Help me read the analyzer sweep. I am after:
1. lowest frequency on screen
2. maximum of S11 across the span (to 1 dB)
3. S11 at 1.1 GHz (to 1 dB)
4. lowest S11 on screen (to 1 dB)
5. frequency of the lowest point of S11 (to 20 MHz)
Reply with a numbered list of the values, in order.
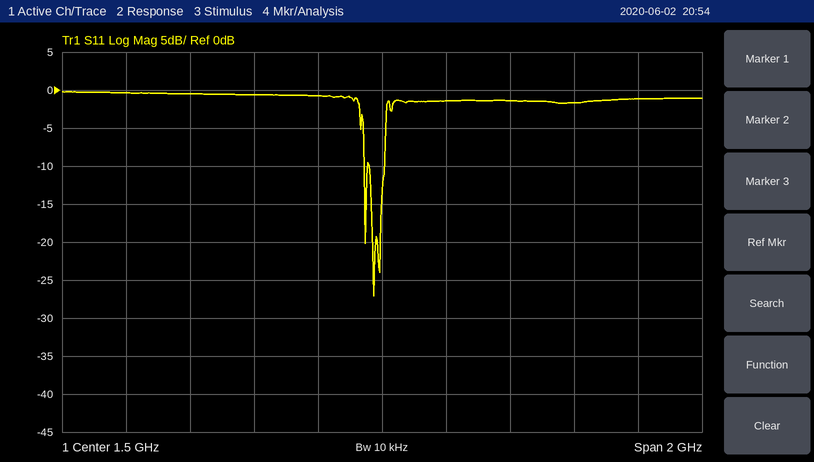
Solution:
1. 500 MHz
2. 0 dB
3. -1 dB
4. -27 dB
5. 1.48 GHz
